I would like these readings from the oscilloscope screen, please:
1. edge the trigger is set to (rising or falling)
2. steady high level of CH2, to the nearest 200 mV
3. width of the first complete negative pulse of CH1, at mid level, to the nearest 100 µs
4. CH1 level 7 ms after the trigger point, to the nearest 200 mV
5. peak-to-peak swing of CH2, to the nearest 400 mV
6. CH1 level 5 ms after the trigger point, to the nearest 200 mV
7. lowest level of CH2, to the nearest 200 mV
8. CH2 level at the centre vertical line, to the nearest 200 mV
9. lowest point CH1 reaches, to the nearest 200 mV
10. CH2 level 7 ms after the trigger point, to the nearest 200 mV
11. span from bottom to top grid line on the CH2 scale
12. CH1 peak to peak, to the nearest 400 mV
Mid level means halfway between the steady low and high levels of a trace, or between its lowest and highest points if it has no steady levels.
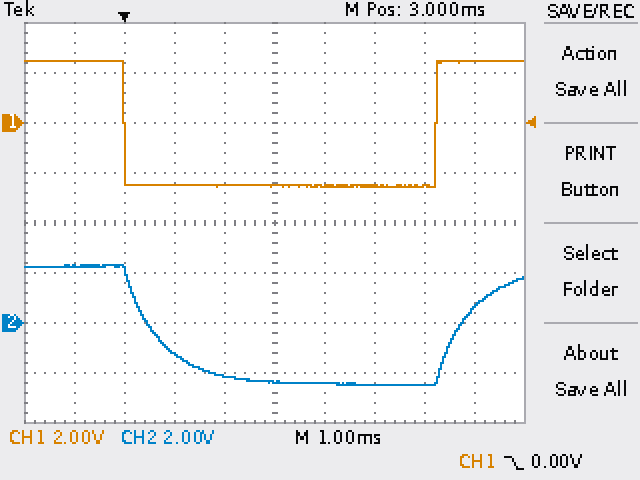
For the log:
falling
2.2 V
6.2 ms
2.4 V
4.8 V
-2.6 V
-2.4 V
-2.4 V
-2.6 V
600 mV
16 V
5.2 V
